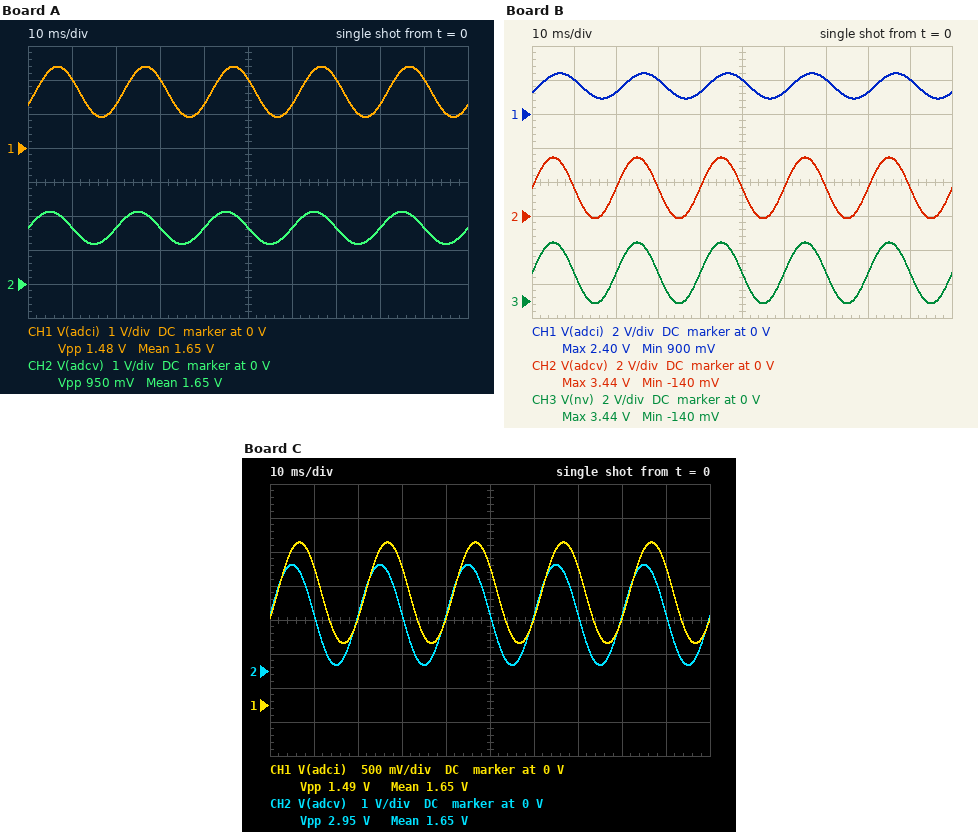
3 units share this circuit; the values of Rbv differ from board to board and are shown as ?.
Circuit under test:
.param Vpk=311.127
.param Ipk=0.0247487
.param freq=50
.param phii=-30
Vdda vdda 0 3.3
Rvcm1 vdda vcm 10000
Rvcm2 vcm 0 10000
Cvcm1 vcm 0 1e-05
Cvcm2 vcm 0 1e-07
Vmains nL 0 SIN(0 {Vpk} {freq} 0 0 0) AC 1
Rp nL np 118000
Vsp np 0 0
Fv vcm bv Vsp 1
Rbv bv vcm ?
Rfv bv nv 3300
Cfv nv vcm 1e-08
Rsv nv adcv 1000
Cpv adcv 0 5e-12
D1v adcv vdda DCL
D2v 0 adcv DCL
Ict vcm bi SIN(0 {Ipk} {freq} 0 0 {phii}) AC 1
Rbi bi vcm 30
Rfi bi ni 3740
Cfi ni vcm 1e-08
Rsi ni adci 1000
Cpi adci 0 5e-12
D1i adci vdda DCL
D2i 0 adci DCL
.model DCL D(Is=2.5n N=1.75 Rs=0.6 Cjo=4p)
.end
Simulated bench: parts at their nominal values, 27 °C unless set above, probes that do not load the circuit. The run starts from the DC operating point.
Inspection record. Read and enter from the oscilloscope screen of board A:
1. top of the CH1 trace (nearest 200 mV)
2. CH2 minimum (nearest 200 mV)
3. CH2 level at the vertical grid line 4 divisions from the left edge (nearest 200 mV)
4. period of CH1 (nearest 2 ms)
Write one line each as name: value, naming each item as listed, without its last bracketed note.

top of the CH1 trace: 2.4 V
CH2 minimum: 1.2 V
CH2 level at the vertical grid line 4 divisions from the left edge: 1.6 V
period of CH1: 20 ms
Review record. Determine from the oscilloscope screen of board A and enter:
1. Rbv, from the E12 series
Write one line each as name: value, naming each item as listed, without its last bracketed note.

Rbv, from the E12 series: 180 Ω
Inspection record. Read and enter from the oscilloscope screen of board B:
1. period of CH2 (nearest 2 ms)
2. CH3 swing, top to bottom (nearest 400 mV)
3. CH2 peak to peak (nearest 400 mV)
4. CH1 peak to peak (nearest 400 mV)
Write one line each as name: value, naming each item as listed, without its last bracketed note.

period of CH2: 20 ms
CH3 swing, top to bottom: 3.6 V
CH2 peak to peak: 3.6 V
CH1 peak to peak: 1.6 V
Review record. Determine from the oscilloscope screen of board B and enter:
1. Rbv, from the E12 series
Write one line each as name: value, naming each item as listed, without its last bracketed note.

Rbv, from the E12 series: 680 Ω
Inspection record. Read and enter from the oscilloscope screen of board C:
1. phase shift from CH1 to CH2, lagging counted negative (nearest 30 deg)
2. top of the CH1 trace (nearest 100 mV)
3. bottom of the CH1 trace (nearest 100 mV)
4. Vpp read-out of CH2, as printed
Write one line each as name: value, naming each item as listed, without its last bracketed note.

phase shift from CH1 to CH2, lagging counted negative: 30 deg
top of the CH1 trace: 2.4 V
bottom of the CH1 trace: 900 mV
Vpp read-out of CH2, as printed: 2.95 V
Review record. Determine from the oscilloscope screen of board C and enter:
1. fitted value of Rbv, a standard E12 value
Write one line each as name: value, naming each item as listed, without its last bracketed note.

fitted value of Rbv, a standard E12 value: 560 Ω
